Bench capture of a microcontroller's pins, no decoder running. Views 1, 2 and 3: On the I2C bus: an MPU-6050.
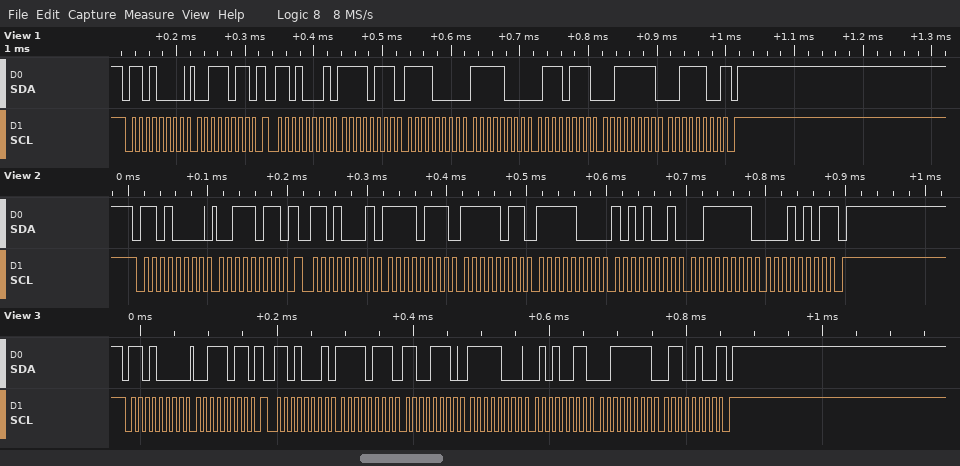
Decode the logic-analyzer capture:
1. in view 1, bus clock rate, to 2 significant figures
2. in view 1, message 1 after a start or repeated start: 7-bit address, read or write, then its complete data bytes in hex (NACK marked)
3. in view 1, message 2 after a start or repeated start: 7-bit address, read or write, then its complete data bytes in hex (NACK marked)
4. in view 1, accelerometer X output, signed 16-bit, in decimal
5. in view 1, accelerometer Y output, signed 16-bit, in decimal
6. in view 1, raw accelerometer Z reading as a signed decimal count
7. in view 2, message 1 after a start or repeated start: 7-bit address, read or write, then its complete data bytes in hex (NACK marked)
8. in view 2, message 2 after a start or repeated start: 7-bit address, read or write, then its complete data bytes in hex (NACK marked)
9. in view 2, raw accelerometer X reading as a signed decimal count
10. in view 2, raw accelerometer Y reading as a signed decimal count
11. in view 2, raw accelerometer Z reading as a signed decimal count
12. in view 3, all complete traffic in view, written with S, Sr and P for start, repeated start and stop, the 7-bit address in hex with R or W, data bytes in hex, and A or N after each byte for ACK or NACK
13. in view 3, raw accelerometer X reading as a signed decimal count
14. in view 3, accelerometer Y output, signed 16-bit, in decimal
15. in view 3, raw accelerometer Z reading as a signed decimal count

100 kHz
0x68 write: 3B
0x68 read: F7 F0 F8 77 3F 3C NACK
-2064
-1929
16188
0x68 write: 3B
0x68 read: F7 FB F8 A9 3F 15 NACK
-2053
-1879
16149
S 68W A 3B A Sr 68R A F7 A CE A F8 A 53 A 3F A 64 N P
-2098
-1965
16228
